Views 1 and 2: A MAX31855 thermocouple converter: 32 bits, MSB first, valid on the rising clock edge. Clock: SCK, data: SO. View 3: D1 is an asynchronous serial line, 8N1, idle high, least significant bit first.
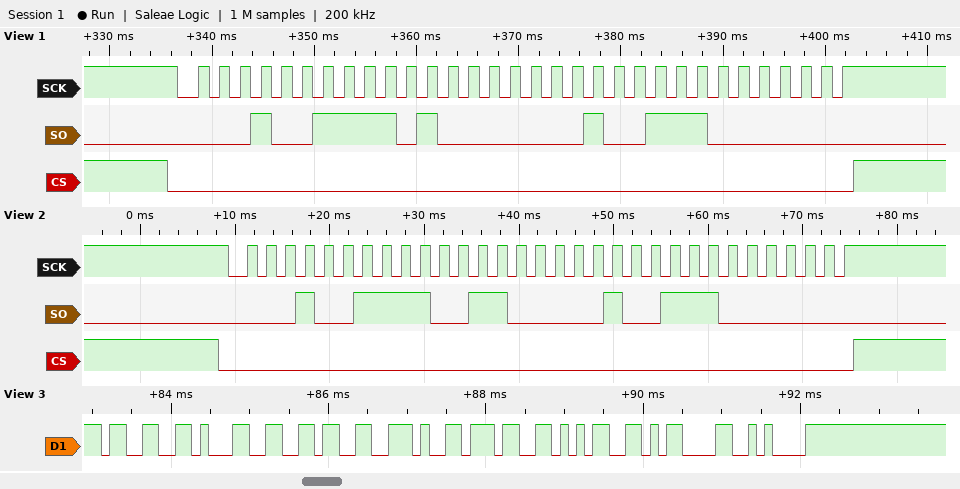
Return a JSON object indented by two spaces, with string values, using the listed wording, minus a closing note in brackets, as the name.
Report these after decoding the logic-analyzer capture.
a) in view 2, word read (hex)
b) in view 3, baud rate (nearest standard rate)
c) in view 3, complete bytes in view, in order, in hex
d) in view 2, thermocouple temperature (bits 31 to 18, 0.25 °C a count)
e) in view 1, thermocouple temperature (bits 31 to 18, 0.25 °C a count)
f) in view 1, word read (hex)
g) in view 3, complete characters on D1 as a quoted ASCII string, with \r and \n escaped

{
  "in view 2, word read": "0x13CC1380",
  "in view 3, baud rate": "9600 baud",
  "in view 3, complete bytes in view, in order, in hex": "33 31 36 2E 37 35 0D 0A",
  "in view 2, thermocouple temperature": "316.75 °C",
  "in view 1, thermocouple temperature": "317.00 °C",
  "in view 1, word read": "0x13D01380",
  "in view 3, complete characters on D1 as a quoted ASCII string, with \\r and \\n escaped": "\"316.75\\r\\n\""
}
